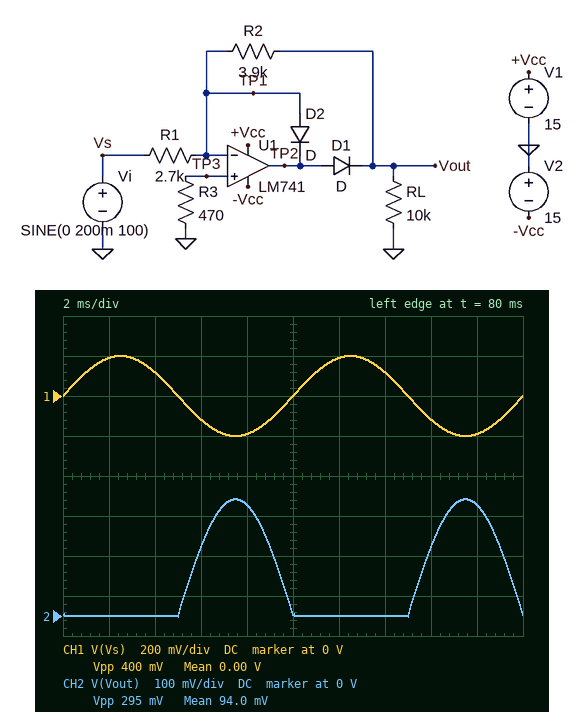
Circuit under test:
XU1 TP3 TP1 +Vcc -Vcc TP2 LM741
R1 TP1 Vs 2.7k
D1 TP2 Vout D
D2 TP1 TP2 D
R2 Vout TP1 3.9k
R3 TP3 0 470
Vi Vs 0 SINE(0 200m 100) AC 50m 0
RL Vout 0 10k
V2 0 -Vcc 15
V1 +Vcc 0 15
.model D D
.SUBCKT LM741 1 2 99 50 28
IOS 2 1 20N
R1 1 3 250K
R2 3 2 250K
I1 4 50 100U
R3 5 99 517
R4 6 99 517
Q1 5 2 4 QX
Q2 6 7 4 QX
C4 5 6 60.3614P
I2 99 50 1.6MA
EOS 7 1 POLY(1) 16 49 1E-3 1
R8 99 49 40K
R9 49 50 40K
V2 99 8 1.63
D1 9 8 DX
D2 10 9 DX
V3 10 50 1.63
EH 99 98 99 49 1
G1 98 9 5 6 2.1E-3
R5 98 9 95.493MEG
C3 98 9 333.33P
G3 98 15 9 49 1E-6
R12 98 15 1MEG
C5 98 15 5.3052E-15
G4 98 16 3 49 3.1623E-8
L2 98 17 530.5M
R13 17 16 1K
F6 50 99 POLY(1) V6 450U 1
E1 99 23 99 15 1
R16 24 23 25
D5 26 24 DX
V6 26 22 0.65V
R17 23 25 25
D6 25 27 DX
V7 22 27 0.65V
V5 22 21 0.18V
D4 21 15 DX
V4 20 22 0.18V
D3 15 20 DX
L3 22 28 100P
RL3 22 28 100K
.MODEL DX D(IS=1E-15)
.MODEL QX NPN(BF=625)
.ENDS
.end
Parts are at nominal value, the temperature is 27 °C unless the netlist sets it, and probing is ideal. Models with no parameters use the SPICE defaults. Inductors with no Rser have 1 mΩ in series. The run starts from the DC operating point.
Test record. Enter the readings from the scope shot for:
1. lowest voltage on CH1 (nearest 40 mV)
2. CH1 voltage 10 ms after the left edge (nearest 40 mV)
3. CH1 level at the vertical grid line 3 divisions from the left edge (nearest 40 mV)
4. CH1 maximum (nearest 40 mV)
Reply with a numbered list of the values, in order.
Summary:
1. -200 mV
2. 0 V
3. -120 mV
4. 200 mV
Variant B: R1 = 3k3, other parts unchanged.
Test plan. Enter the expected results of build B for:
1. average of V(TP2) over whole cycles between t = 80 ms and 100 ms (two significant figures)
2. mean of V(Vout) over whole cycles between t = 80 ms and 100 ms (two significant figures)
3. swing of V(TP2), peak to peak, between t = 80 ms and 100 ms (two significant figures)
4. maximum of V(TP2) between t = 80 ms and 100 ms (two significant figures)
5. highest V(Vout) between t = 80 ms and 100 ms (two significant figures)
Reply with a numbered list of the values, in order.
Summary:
1. 84 mV
2. 77 mV
3. 1.4 V
4. 830 mV
5. 240 mV
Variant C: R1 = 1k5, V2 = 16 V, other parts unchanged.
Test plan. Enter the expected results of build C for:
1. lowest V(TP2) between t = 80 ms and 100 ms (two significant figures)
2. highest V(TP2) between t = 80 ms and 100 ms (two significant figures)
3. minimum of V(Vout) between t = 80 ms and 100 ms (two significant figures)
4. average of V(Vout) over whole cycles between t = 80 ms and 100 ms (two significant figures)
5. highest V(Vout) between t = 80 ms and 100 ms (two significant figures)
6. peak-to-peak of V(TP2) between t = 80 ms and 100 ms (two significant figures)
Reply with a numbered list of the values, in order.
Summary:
1. -600 mV
2. 1.1 V
3. -3.1 mV
4. 170 mV
5. 520 mV
6. 1.7 V
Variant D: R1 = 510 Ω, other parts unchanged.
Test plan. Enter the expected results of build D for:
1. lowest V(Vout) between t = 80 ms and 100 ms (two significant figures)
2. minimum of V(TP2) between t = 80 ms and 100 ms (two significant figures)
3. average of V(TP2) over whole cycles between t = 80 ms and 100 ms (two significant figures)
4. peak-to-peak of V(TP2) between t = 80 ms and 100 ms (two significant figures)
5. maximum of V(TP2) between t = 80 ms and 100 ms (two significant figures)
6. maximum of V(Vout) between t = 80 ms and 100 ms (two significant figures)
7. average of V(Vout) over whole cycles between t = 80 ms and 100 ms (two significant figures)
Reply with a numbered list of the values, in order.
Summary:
1. -3.3 mV
2. -630 mV
3. 500 mV
4. 2.8 V
5. 2.2 V
6. 1.5 V
7. 490 mV
